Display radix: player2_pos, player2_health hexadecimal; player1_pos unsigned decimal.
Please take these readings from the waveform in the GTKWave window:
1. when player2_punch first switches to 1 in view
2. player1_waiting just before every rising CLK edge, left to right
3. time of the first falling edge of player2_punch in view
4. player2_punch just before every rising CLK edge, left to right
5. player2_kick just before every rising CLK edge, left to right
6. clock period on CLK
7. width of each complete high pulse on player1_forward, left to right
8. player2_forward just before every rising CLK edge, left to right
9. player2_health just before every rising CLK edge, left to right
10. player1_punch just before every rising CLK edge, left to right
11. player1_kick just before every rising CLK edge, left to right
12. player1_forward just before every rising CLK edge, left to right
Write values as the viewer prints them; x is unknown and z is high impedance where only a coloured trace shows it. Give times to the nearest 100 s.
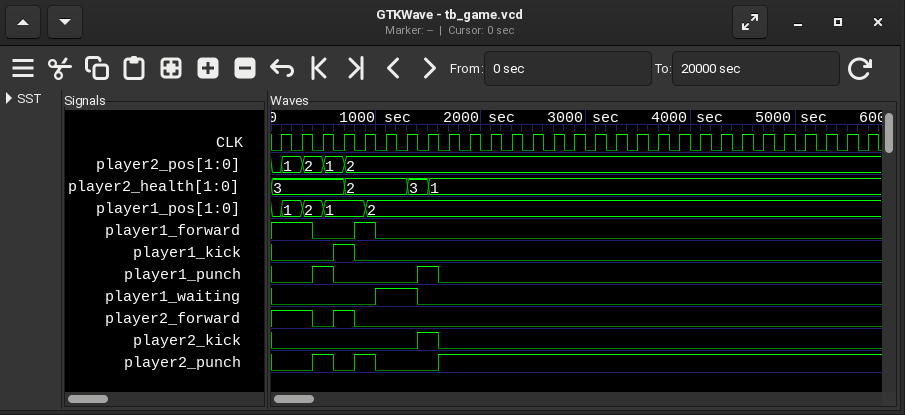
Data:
400 s
0 0 0 0 0 1 1 0 0 0 0 0 0 0 0 0 0 0 0 0 0 0 0 0 0 0 0 0 0
600 s
0 0 1 0 1 0 0 0 1 1 1 1 1 1 1 1 1 1 1 1 1 1 1 1 1 1 1 1 1
0 0 0 0 0 0 0 1 0 0 0 0 0 0 0 0 0 0 0 0 0 0 0 0 0 0 0 0 0
200 s
200 s
1 1 0 1 0 0 0 0 0 0 0 0 0 0 0 0 0 0 0 0 0 0 0 0 0 0 0 0 0
3, 3, 3, 3, 2, 2, 2, 3, 1, 1, 1, 1, 1, 1, 1, 1, 1, 1, 1, 1, 1, 1, 1, 1, 1, 1, 1, 1, 1
0 0 1 0 0 0 0 1 0 0 0 0 0 0 0 0 0 0 0 0 0 0 0 0 0 0 0 0 0
0 0 0 1 0 0 0 0 0 0 0 0 0 0 0 0 0 0 0 0 0 0 0 0 0 0 0 0 0
1 1 0 0 1 0 0 0 0 0 0 0 0 0 0 0 0 0 0 0 0 0 0 0 0 0 0 0 0
